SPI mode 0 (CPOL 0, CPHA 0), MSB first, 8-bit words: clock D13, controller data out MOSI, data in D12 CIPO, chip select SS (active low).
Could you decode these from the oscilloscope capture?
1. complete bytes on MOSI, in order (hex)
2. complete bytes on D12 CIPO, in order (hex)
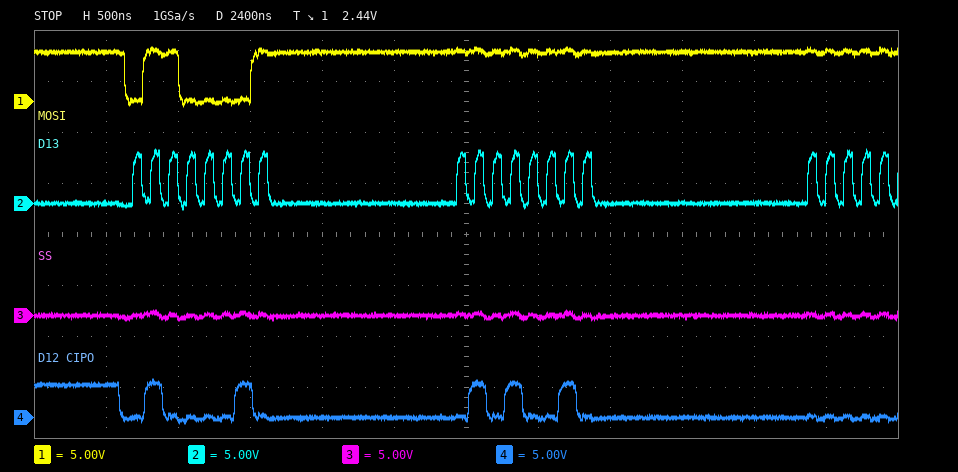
61 FF
42 52
